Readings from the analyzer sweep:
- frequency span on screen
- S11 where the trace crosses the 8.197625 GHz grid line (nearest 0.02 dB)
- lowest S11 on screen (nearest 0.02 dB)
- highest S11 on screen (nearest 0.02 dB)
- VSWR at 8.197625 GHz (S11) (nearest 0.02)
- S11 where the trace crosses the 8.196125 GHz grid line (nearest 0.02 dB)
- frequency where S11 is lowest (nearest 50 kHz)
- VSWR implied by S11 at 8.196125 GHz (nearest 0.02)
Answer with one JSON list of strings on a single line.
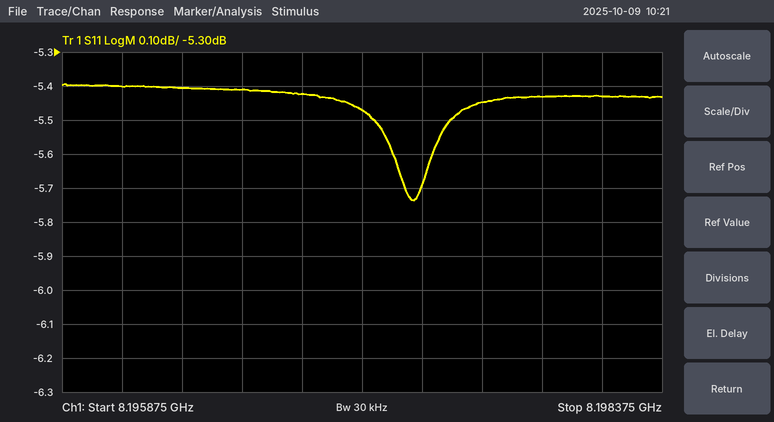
["2.5 MHz", "-5.44 dB", "-5.74 dB", "-5.40 dB", "3.30", "-5.40 dB", "8.19735 GHz", "3.32"]
